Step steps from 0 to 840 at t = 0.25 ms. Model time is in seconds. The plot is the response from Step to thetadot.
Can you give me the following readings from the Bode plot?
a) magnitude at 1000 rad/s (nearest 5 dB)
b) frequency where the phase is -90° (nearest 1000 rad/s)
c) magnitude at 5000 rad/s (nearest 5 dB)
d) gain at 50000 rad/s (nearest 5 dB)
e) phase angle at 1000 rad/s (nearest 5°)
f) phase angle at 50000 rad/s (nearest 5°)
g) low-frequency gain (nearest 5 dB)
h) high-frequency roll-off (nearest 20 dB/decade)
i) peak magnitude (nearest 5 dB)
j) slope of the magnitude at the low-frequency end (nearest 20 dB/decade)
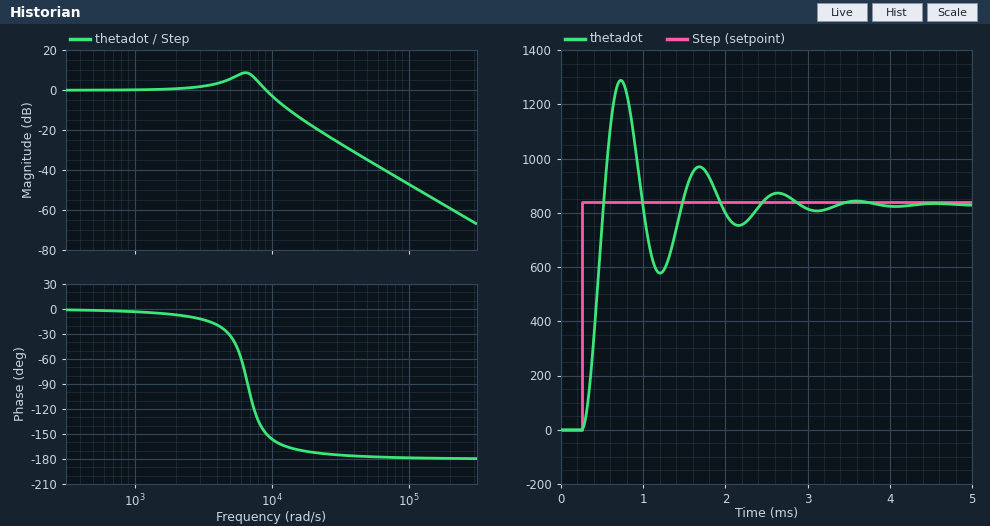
0 dB
7000 rad/s
5 dB
-35 dB
-5°
-175°
0 dB
-40 dB/decade
10 dB
0 dB/decade
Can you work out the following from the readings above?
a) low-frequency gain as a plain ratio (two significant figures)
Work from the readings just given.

1.0
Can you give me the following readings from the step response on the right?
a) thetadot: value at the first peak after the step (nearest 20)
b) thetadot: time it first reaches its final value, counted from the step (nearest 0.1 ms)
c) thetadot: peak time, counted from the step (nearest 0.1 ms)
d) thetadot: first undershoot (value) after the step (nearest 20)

1280
0.3 ms
0.5 ms
580
